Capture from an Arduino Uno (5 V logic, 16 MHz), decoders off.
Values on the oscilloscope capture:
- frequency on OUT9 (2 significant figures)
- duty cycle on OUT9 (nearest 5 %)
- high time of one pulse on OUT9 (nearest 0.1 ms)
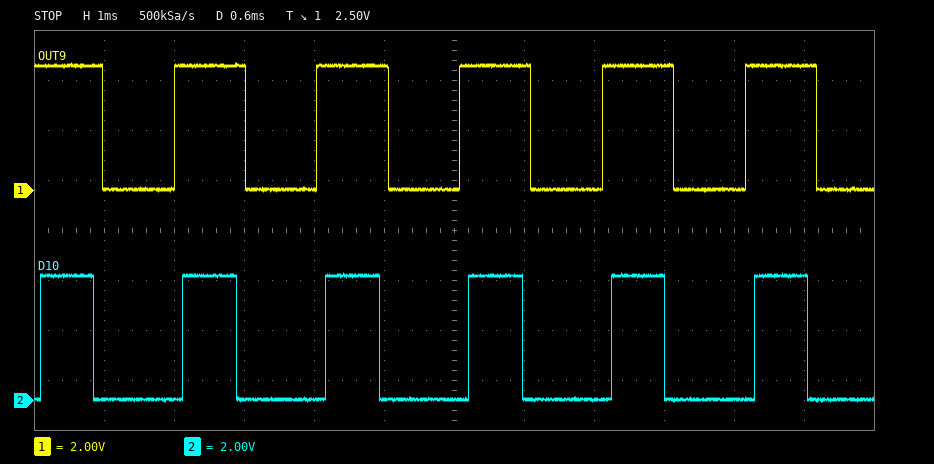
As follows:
490 Hz
50 %
1.0 ms
